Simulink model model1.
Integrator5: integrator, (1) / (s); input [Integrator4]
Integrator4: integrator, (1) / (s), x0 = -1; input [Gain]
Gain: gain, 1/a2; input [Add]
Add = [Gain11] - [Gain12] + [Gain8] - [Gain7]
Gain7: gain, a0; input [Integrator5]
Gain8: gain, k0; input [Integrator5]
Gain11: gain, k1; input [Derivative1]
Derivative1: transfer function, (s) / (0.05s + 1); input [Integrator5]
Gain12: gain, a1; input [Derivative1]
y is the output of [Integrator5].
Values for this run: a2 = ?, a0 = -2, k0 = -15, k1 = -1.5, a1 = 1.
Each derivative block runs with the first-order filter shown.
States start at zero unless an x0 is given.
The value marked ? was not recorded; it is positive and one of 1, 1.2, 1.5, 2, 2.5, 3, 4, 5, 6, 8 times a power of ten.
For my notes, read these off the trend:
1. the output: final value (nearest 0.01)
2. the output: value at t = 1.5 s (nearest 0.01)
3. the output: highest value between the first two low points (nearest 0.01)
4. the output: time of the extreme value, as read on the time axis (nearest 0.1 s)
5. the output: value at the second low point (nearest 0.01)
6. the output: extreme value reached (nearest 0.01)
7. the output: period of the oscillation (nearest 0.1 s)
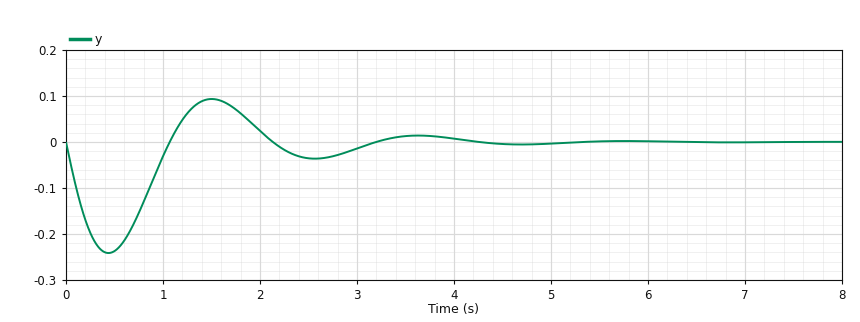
0.00
0.09
0.09
0.4 s
-0.04
-0.24
2.1 s
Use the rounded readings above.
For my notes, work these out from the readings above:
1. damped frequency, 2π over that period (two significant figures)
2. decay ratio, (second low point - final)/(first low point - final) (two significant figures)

3.0 rad/s
0.17
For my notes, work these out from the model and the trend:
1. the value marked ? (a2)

1.5
